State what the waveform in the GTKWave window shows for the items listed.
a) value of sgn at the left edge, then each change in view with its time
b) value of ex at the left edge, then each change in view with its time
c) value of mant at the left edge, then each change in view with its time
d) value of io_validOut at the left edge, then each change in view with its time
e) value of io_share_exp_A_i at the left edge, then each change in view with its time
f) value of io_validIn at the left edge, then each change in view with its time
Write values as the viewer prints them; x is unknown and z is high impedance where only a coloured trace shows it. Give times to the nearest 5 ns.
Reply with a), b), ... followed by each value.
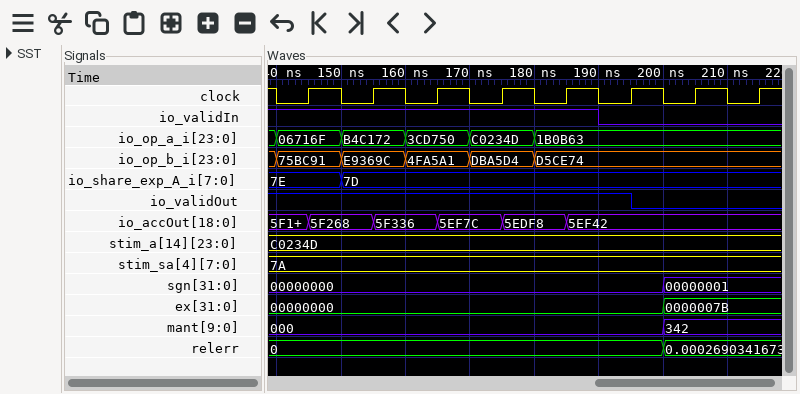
a) 00000000, 00000001 at 200 ns
b) 00000000, 0000007B at 200 ns
c) 000, 342 at 200 ns
d) 1, 0 at 195 ns
e) 7E, 7D at 150 ns
f) 1, 0 at 190 ns
